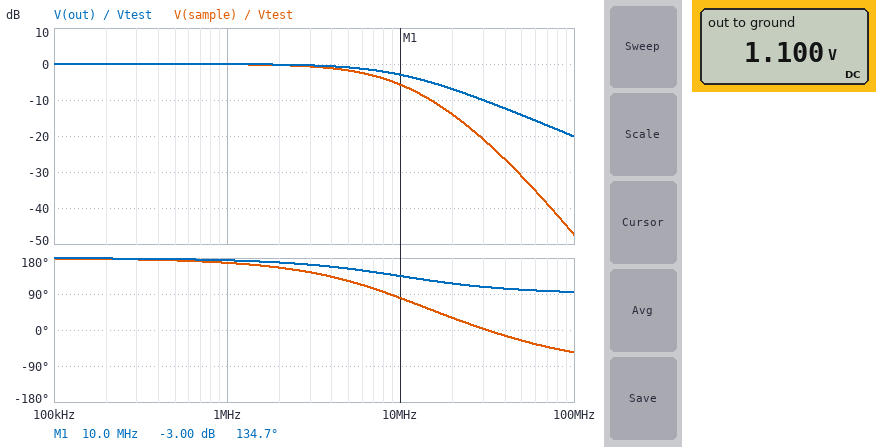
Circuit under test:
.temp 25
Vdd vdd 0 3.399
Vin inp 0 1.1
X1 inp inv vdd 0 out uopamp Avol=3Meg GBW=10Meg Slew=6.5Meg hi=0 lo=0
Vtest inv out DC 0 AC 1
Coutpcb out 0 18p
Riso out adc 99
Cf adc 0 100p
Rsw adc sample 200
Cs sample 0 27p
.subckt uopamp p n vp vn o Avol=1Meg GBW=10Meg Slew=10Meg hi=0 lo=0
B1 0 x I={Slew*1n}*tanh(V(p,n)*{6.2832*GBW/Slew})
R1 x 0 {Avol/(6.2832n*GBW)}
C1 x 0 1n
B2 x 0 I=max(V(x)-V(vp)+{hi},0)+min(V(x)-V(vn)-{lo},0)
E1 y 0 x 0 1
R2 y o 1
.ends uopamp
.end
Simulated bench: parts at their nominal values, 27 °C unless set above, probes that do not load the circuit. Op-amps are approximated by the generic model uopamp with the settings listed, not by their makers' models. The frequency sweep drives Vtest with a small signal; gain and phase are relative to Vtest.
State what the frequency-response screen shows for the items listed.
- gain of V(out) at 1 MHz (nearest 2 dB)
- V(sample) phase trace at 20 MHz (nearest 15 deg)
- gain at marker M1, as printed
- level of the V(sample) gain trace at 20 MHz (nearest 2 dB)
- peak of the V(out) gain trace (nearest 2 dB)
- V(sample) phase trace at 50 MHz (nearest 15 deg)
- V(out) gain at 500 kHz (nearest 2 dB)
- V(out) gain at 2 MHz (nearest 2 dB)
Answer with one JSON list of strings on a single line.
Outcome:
["0 dB", "30 deg", "-3.00 dB", "-14 dB", "0 dB", "-30 deg", "0 dB", "0 dB"]
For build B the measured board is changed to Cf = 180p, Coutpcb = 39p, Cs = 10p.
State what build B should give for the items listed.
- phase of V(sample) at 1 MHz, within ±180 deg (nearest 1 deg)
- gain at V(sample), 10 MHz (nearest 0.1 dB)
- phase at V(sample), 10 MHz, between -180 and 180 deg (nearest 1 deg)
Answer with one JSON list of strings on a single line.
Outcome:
["167 deg", "-6.9 dB", "78 deg"]
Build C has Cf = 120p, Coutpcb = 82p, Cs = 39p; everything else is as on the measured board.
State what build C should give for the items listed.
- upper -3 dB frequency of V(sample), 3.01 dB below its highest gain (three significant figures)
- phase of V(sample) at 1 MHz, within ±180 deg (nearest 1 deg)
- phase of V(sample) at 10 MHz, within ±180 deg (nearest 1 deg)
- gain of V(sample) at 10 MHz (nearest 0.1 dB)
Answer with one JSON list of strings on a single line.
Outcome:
["5.80 MHz", "166 deg", "68 deg", "-7.1 dB"]
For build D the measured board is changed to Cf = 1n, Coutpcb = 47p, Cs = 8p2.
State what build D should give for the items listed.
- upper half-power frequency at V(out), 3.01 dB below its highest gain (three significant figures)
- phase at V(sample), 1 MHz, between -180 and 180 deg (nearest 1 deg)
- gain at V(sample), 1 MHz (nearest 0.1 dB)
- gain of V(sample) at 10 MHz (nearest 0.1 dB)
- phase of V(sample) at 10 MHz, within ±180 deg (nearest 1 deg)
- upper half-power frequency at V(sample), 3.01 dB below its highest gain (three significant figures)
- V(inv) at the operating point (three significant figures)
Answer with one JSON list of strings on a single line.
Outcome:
["9.95 MHz", "142 deg", "-1.5 dB", "-19.1 dB", "48 deg", "1.56 MHz", "1.10 V"]
